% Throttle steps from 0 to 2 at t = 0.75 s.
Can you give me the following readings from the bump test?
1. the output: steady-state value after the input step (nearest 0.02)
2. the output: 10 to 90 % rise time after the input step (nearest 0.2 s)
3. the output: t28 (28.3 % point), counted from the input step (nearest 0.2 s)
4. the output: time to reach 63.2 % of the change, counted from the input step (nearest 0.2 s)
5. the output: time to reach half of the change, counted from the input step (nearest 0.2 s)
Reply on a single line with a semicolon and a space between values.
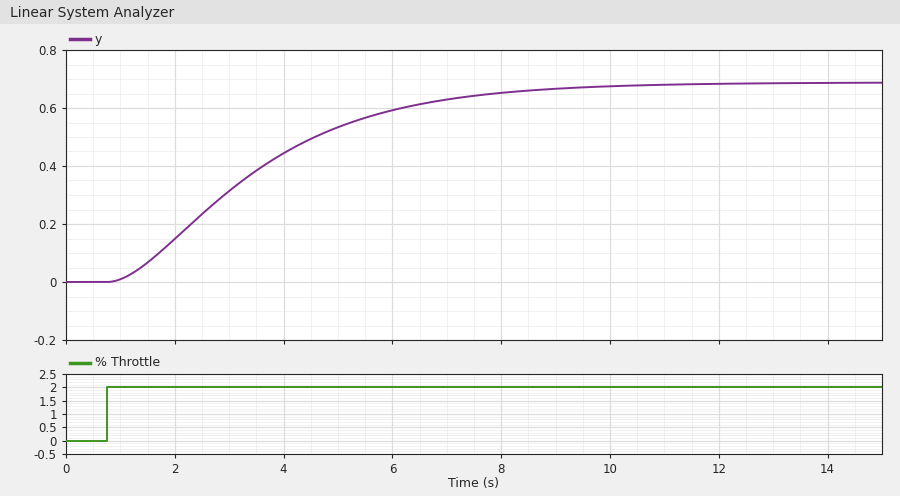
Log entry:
0.68; 5.2 s; 1.6 s; 3.2 s; 2.4 s
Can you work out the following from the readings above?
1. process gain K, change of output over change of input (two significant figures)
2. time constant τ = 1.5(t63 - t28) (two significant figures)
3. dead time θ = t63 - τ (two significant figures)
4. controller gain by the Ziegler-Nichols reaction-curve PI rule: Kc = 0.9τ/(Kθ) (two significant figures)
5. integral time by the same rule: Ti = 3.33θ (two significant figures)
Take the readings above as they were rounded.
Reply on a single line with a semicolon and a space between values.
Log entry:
0.34; 2.4 s; 0.80 s; 7.9; 2.7 s
